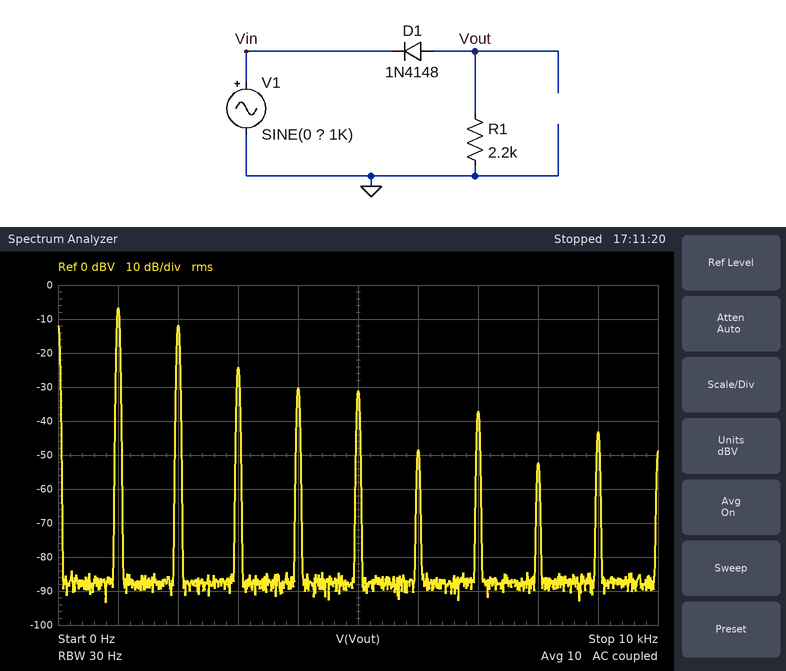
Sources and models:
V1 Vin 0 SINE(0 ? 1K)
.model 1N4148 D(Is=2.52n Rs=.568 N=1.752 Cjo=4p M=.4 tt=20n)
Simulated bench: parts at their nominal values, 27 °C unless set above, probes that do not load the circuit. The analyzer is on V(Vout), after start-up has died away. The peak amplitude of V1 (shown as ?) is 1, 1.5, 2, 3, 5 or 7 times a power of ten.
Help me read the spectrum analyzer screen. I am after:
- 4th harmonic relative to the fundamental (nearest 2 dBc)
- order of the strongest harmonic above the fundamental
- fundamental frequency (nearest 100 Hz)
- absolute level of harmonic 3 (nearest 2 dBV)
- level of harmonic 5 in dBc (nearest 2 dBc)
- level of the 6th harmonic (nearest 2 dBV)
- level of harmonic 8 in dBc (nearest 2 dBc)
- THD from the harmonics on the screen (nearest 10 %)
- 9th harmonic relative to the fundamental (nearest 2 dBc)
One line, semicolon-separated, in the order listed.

-24 dBc; 2; 1.0 kHz; -24 dBV; -24 dBc; -48 dBV; -46 dBc; 60 %; -36 dBc
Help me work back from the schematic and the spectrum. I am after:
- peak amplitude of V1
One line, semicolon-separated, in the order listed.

2 V
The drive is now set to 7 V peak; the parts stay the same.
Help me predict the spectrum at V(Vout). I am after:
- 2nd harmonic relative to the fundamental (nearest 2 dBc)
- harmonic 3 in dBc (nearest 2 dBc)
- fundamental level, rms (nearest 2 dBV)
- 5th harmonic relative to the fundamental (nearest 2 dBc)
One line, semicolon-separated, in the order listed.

-6 dBc; -28 dBc; 6 dBV; -34 dBc
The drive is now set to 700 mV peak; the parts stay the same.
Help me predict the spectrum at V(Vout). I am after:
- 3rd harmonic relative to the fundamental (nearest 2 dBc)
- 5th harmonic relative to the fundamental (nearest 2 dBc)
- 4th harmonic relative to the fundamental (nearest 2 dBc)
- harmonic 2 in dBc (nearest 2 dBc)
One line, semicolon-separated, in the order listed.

-8 dBc; -38 dBc; -18 dBc; -2 dBc
